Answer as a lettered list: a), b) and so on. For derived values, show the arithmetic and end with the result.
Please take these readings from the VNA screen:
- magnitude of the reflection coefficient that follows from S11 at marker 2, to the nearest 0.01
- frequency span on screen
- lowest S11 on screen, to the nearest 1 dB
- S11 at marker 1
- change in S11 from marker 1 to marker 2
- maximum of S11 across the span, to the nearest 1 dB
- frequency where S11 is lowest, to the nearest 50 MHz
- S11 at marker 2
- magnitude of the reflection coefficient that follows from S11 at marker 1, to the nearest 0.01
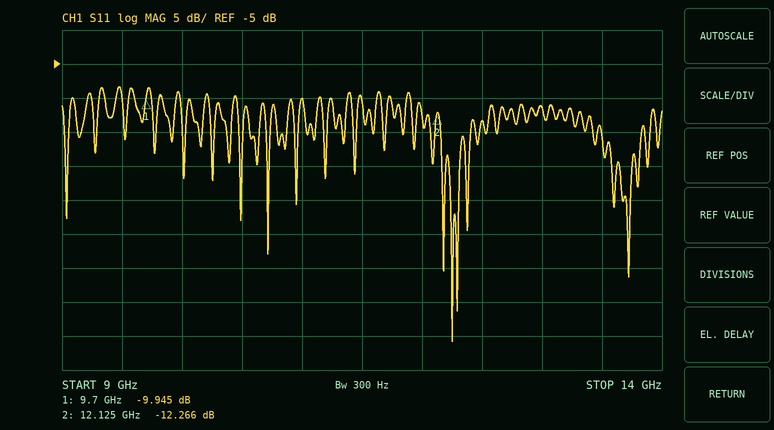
a) 10^(-12.266/20) ≈ 0.24
b) 5 GHz
c) -46 dB
d) -9.945 dB
e) -12.266 − (-9.945) = -2.321 dB
f) -8 dB
g) 12.25 GHz
h) -12.266 dB
i) 10^(-9.945/20) ≈ 0.32
